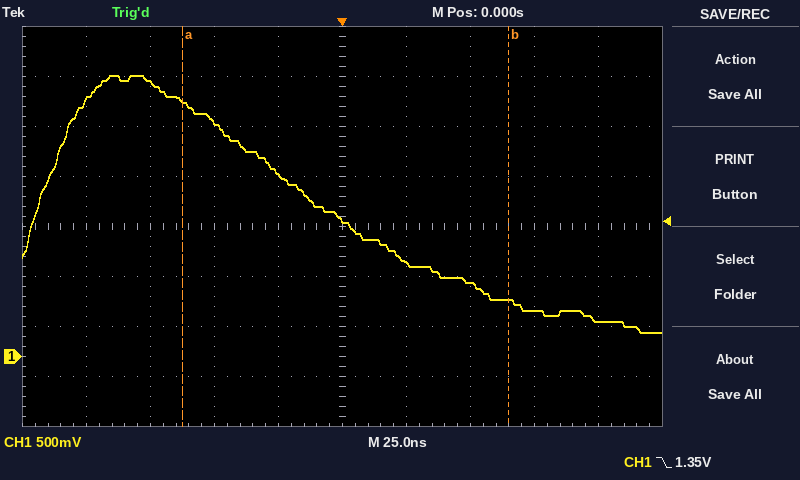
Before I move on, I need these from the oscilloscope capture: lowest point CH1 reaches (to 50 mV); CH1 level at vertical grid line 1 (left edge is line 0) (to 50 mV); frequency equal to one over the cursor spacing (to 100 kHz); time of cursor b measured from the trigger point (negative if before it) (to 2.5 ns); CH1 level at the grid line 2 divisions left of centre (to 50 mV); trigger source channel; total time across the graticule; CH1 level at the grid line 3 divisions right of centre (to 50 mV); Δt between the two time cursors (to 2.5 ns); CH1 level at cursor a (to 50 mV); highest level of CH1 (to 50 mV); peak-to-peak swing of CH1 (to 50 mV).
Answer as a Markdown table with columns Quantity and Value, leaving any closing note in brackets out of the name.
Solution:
| Quantity | Value |
|---|---|
| lowest point CH1 reaches | 250 mV |
| CH1 level at vertical grid line 1 (left edge is line 0) | 2.55 V |
| frequency equal to one over the cursor spacing | 7.8 MHz |
| time of cursor b measured from the trigger point (negative if before it) | +65.0 ns |
| CH1 level at the grid line 2 divisions left of centre | 2.35 V |
| trigger source channel | CH1 |
| total time across the graticule | 250 ns |
| CH1 level at the grid line 3 divisions right of centre | 450 mV |
| Δt between the two time cursors | 127.5 ns |
| CH1 level at cursor a | 2.55 V |
| highest level of CH1 | 2.80 V |
| peak-to-peak swing of CH1 | 2.55 V |
